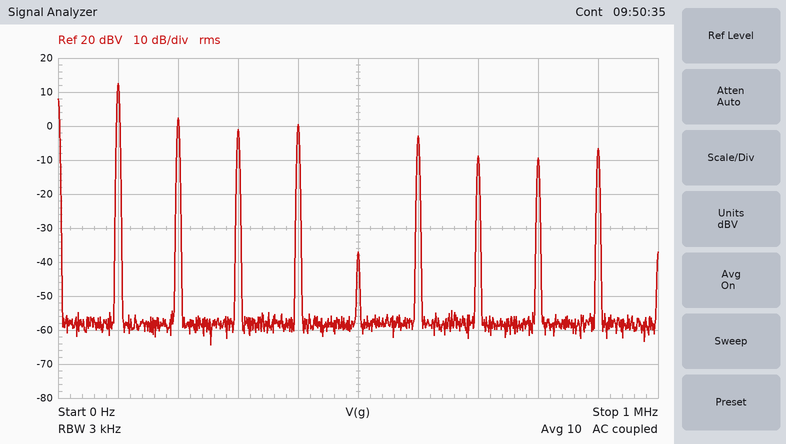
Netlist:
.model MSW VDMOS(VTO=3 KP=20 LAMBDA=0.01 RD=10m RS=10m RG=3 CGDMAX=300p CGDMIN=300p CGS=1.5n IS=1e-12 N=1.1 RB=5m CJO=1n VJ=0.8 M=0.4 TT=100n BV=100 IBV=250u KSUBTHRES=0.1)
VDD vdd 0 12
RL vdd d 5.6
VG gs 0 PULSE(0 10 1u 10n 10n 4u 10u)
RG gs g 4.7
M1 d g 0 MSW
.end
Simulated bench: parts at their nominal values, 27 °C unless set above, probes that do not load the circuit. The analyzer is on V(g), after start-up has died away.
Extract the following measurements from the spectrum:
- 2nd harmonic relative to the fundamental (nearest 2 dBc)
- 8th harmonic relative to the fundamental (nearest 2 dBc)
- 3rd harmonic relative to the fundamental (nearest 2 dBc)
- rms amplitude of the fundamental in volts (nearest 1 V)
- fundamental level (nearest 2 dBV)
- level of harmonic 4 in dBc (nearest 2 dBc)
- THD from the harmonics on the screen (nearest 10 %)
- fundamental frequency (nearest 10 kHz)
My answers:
-10 dBc
-22 dBc
-14 dBc
4 V
12 dBV
-12 dBc
50 %
100 kHz
